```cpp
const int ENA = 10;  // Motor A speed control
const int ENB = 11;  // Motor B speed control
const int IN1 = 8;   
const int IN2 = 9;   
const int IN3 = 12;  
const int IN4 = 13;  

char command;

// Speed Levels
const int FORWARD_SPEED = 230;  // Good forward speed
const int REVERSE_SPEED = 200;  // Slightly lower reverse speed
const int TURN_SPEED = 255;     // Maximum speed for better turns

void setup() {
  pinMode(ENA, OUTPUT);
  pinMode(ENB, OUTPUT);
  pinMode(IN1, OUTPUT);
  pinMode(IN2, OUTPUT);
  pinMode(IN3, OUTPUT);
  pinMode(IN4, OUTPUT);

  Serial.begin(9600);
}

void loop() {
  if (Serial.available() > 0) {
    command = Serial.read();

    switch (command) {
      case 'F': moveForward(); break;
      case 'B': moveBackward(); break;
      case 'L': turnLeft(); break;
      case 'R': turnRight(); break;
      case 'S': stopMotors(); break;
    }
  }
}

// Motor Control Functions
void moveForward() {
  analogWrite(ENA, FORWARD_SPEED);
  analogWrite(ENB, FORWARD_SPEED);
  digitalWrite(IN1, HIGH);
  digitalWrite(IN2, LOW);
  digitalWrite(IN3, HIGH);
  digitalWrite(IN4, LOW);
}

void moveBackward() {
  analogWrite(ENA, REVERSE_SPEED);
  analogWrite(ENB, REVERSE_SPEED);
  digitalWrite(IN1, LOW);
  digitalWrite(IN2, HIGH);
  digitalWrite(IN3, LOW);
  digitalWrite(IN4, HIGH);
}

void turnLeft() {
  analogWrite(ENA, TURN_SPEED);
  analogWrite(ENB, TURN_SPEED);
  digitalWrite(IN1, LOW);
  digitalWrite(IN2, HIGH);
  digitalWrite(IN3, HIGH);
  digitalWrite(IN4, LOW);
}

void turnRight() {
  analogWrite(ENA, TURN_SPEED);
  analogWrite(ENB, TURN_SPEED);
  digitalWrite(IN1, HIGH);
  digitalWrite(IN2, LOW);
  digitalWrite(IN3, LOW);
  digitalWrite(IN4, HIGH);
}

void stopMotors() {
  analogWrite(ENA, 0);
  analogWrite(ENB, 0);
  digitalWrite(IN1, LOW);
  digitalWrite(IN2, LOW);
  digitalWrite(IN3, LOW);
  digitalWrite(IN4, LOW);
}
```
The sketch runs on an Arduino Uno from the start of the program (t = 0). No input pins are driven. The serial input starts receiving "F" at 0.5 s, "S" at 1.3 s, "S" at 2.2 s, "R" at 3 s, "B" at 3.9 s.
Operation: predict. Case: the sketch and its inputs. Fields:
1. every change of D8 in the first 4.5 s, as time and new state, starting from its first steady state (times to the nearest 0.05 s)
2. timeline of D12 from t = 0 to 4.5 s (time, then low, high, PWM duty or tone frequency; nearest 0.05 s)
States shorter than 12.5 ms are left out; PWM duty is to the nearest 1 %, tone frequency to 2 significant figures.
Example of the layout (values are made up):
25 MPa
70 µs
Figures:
0 s low; 0.5 s high; 1.3 s low; 3 s high; 3.9 s low
0 s low; 0.5 s high; 1.3 s low
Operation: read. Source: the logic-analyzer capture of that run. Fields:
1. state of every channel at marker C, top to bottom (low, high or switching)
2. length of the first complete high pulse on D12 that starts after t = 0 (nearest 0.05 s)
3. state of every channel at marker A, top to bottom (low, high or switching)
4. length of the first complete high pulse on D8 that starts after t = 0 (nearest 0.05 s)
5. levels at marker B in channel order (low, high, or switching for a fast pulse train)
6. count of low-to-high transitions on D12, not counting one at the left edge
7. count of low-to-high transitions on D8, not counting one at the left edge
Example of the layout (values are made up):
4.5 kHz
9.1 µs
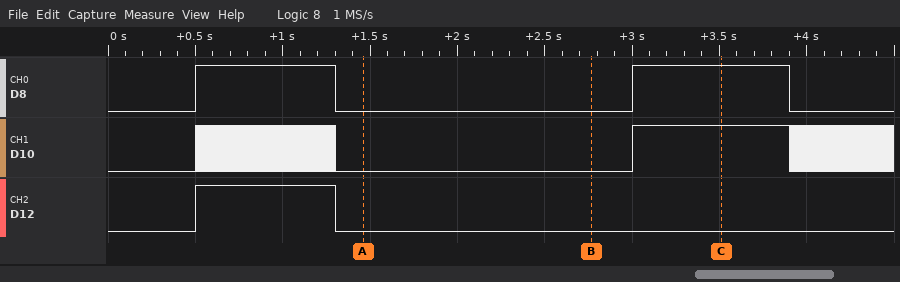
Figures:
D8 high, D10 high, D12 low
0.80 s
D8 low, D10 low, D12 low
0.80 s
D8 low, D10 low, D12 low
1
2
